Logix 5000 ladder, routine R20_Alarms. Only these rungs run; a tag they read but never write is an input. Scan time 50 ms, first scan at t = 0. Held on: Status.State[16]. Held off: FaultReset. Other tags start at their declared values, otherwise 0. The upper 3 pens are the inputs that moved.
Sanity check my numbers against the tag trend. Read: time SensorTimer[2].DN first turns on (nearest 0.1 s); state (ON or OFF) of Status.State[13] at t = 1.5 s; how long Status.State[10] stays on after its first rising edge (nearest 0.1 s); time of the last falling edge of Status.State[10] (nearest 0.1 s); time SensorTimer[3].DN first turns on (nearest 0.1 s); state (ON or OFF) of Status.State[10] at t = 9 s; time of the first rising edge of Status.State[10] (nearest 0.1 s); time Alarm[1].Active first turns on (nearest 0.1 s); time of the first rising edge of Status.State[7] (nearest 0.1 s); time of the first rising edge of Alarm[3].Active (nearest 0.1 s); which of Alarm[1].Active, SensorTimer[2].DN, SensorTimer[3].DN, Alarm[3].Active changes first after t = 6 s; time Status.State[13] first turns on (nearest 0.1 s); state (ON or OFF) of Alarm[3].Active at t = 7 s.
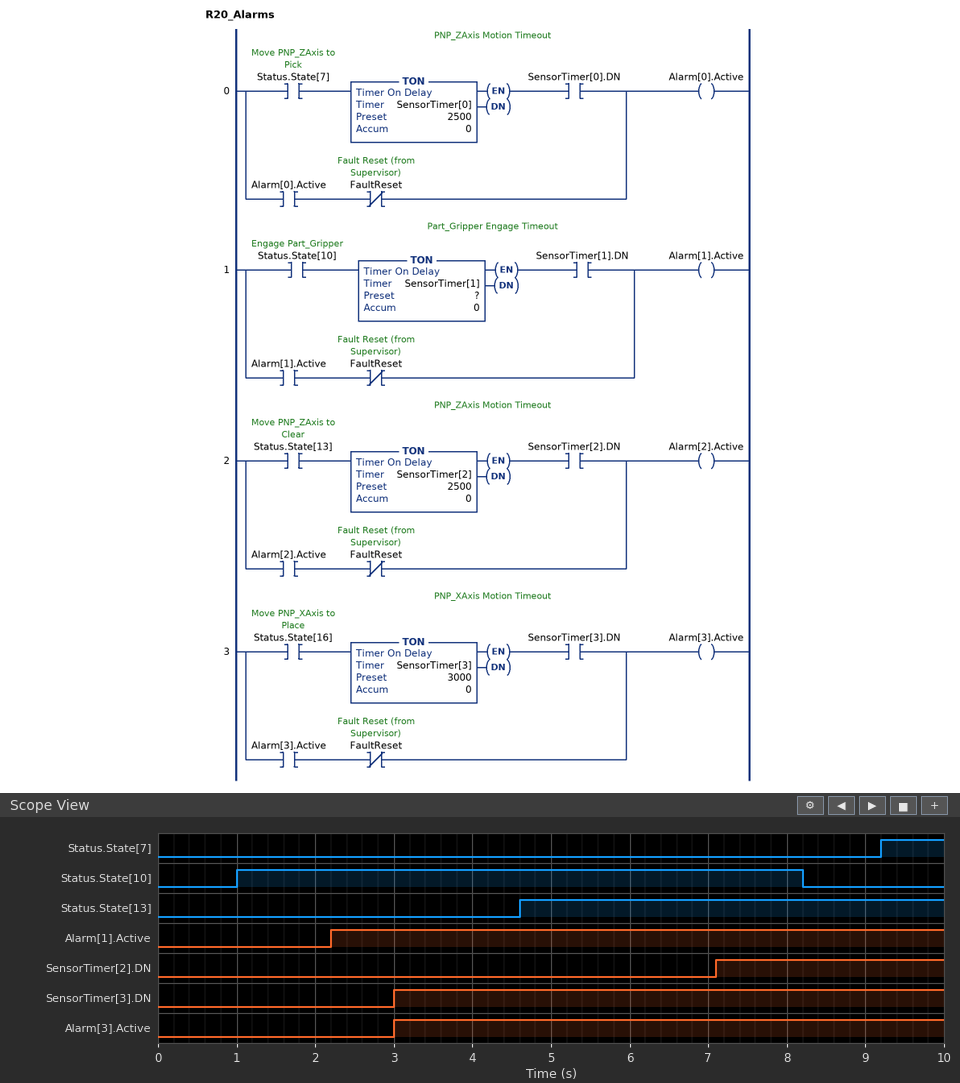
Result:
7.1 s
OFF
7.2 s
8.2 s
3.0 s
OFF
1.0 s
2.2 s
9.2 s
3.0 s
SensorTimer[2].DN
4.6 s
ON
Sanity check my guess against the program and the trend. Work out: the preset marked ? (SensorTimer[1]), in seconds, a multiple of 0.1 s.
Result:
1.2 s
